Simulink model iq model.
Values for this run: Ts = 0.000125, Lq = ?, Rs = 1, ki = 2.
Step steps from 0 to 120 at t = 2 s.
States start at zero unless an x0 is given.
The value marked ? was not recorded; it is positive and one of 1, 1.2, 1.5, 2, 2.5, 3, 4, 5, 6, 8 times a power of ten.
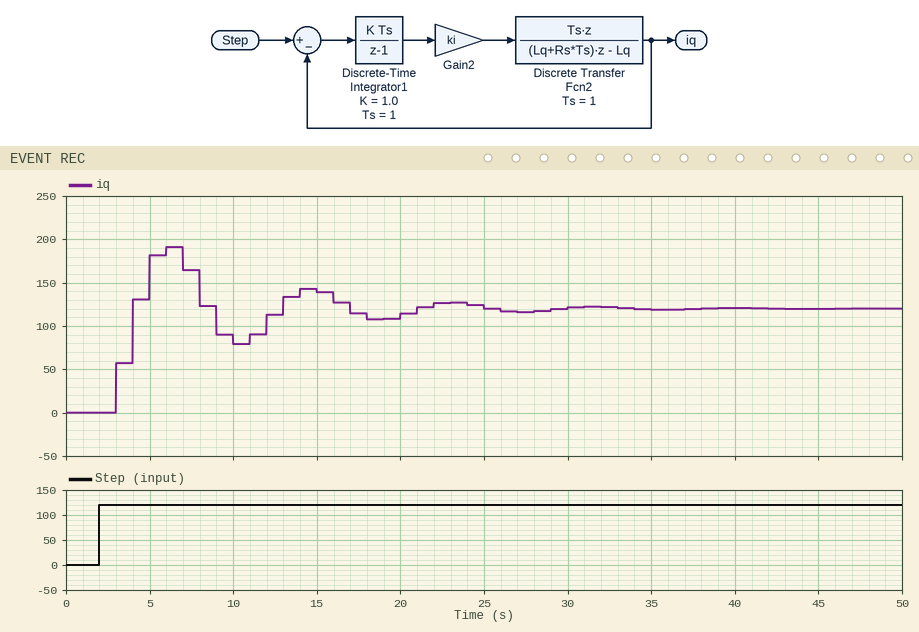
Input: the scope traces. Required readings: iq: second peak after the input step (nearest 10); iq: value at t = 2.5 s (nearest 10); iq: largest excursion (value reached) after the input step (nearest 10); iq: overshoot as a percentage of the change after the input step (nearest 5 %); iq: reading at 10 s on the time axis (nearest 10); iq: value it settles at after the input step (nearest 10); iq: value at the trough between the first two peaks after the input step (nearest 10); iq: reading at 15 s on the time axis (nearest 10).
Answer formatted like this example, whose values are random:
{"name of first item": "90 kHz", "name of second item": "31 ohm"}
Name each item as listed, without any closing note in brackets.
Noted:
{"iq: second peak after the input step": "140", "iq: value at t = 2.5 s": "0", "iq: largest excursion (value reached) after the input step": "190", "iq: overshoot as a percentage of the change after the input step": "60 %", "iq: reading at 10 s on the time axis": "80", "iq: value it settles at after the input step": "120", "iq: value at the trough between the first two peaks after the input step": "80", "iq: reading at 15 s on the time axis": "140"}
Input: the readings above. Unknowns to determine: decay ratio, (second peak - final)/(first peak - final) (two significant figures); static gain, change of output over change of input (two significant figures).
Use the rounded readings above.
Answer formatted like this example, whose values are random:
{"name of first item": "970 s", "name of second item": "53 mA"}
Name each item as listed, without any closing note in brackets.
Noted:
{"decay ratio, (second peak - final)/(first peak - final)": "0.29", "static gain, change of output over change of input": "1.0"}
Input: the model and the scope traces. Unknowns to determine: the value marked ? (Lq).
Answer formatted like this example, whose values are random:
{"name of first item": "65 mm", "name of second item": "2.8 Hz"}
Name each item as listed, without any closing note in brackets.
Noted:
{"the value marked ?": "0.0004"}
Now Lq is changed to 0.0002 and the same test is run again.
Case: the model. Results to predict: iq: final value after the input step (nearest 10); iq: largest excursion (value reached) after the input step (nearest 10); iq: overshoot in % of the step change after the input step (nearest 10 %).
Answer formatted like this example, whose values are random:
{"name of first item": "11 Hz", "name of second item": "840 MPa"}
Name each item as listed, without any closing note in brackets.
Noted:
{"iq: final value after the input step": "120", "iq: largest excursion (value reached) after the input step": "180", "iq: overshoot in % of the step change after the input step": "50 %"}
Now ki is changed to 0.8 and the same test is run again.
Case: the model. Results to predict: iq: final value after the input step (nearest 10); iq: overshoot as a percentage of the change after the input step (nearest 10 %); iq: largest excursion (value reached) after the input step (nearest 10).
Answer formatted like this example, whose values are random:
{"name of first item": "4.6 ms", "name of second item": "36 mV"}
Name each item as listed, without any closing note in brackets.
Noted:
{"iq: final value after the input step": "120", "iq: overshoot as a percentage of the change after the input step": "40 %", "iq: largest excursion (value reached) after the input step": "170"}
